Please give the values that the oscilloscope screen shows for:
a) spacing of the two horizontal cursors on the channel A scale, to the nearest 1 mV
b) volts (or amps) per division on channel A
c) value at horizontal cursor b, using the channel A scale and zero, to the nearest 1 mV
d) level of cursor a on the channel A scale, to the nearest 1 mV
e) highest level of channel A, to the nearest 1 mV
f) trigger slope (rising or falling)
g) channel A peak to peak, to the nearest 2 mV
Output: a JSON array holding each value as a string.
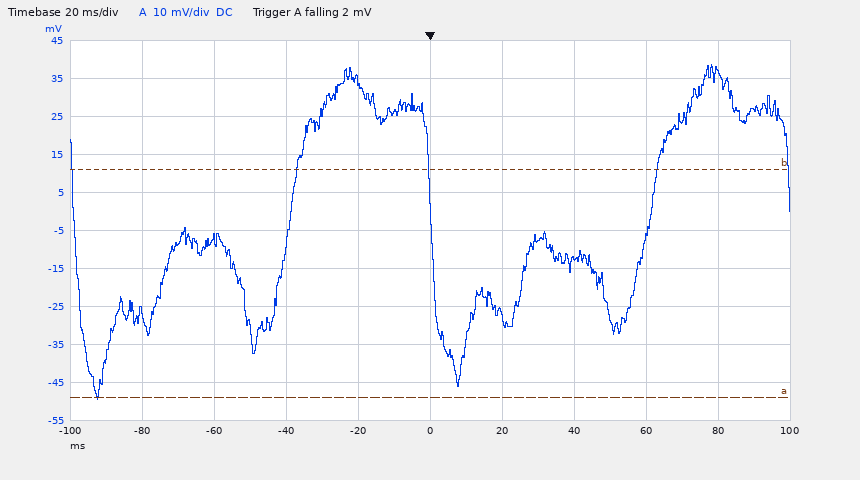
["60 mV", "10 mV", "11 mV", "-49 mV", "39 mV", "falling", "88 mV"]
